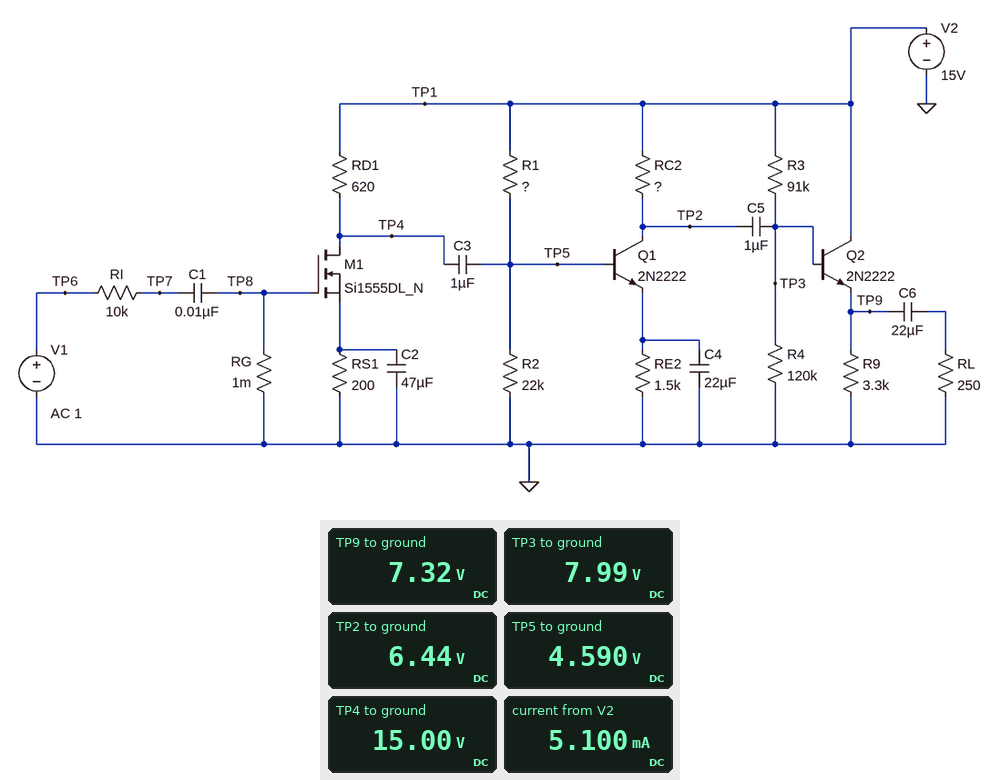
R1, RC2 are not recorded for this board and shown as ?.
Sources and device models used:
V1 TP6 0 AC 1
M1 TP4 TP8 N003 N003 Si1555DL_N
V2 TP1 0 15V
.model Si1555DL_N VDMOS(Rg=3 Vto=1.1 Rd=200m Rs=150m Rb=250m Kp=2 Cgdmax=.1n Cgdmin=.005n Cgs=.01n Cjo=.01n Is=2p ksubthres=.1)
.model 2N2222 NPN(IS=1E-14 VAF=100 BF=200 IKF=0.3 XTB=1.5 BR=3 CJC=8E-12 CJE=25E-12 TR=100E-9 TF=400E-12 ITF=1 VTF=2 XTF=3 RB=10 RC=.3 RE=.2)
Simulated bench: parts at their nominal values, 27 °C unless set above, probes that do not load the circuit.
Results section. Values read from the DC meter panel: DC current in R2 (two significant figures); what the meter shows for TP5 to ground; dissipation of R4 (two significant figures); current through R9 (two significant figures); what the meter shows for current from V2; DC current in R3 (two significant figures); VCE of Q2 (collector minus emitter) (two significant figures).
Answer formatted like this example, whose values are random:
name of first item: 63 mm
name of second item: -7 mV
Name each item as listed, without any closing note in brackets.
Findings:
DC current in R2: 210 µA
what the meter shows for TP5 to ground: 4.590 V
dissipation of R4: 530 µW
current through R9: 2.2 mA
what the meter shows for current from V2: 5.100 mA
DC current in R3: 77 µA
VCE of Q2 (collector minus emitter): 7.7 V
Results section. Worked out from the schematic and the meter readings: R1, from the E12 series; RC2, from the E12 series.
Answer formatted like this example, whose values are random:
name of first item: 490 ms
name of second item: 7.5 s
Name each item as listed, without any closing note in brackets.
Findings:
R1, from the E12 series: 47 kΩ
RC2, from the E12 series: 3.3 kΩ
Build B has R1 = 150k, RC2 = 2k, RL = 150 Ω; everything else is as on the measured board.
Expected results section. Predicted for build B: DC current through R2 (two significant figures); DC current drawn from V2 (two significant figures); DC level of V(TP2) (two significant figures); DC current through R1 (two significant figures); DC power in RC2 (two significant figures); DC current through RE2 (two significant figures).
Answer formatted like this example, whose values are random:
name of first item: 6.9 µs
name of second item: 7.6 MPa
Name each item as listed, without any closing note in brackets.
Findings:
DC current through R2: 84 µA
DC current drawn from V2: 3.2 mA
DC level of V(TP2): 13 V
DC current through R1: 88 µA
DC power in RC2: 1.3 mW
DC current through RE2: 800 µA
